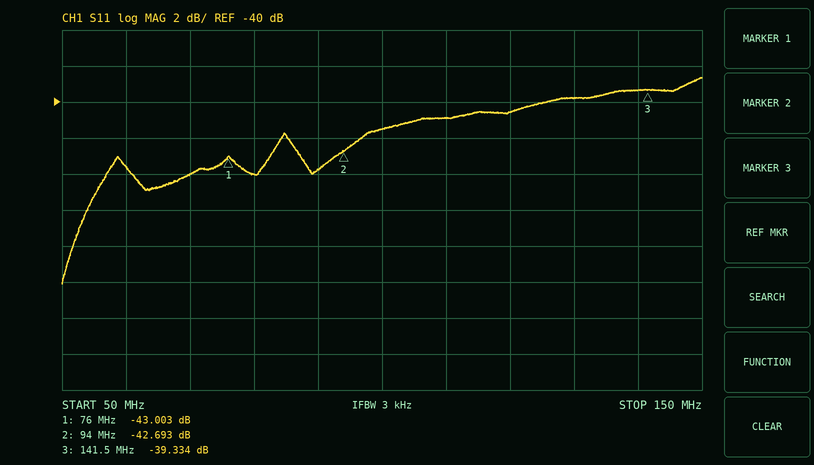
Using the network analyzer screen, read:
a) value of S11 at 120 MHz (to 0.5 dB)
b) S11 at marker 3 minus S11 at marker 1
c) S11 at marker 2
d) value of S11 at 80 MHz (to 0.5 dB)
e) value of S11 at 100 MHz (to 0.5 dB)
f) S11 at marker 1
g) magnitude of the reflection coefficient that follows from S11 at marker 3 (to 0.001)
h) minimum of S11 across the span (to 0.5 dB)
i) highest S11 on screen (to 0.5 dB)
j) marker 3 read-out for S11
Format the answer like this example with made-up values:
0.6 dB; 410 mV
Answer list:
-40.5 dB; 3.669 dB; -42.693 dB; -44.0 dB; -41.5 dB; -43.003 dB; 0.011; -50.0 dB; -38.5 dB; -39.334 dB
